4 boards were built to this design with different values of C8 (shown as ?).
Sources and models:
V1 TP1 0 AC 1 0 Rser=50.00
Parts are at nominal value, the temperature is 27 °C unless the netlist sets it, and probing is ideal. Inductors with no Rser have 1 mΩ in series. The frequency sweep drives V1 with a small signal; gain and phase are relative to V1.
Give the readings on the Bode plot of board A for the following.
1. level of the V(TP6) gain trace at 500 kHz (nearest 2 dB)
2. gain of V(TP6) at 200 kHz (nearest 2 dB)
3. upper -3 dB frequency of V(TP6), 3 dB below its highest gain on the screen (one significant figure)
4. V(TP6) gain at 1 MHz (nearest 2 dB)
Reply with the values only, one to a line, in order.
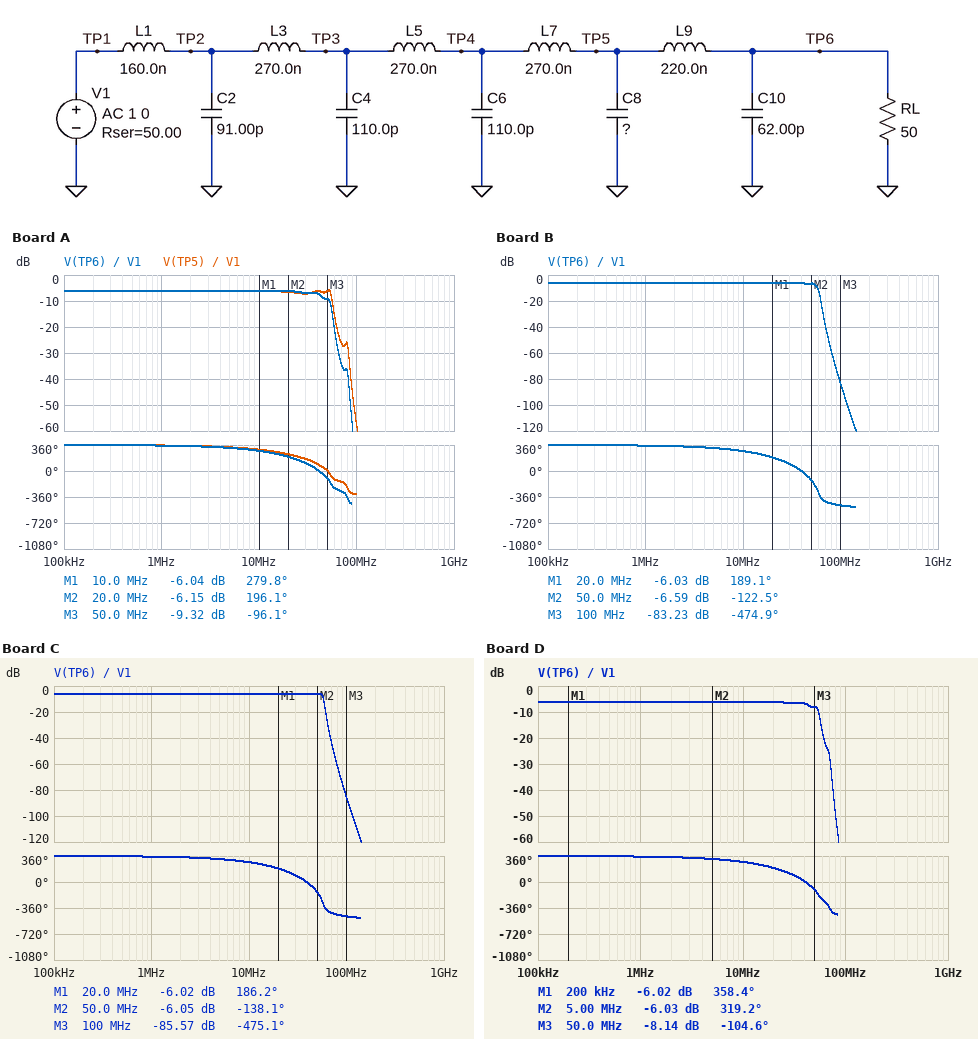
-6 dB
-6 dB
50 MHz
-6 dB
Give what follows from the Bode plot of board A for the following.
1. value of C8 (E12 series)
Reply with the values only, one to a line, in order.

39 pF
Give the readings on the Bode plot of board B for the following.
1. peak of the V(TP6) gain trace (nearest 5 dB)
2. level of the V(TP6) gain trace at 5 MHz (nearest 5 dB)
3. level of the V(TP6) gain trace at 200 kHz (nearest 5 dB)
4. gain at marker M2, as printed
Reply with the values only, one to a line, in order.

-5 dB
-5 dB
-5 dB
-6.59 dB
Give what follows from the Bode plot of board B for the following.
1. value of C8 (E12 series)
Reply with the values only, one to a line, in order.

82 pF
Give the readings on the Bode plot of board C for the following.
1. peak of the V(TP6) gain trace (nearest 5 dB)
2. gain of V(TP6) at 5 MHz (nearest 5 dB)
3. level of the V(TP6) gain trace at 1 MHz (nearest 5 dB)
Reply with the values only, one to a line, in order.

-5 dB
-5 dB
-5 dB
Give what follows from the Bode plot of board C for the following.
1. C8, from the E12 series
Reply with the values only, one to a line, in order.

100 pF
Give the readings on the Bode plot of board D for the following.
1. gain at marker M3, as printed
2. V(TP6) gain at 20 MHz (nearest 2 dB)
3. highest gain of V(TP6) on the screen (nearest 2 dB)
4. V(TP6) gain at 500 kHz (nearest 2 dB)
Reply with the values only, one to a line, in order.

-8.14 dB
-6 dB
-6 dB
-6 dB
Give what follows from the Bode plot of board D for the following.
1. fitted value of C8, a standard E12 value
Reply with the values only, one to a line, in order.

56 pF
